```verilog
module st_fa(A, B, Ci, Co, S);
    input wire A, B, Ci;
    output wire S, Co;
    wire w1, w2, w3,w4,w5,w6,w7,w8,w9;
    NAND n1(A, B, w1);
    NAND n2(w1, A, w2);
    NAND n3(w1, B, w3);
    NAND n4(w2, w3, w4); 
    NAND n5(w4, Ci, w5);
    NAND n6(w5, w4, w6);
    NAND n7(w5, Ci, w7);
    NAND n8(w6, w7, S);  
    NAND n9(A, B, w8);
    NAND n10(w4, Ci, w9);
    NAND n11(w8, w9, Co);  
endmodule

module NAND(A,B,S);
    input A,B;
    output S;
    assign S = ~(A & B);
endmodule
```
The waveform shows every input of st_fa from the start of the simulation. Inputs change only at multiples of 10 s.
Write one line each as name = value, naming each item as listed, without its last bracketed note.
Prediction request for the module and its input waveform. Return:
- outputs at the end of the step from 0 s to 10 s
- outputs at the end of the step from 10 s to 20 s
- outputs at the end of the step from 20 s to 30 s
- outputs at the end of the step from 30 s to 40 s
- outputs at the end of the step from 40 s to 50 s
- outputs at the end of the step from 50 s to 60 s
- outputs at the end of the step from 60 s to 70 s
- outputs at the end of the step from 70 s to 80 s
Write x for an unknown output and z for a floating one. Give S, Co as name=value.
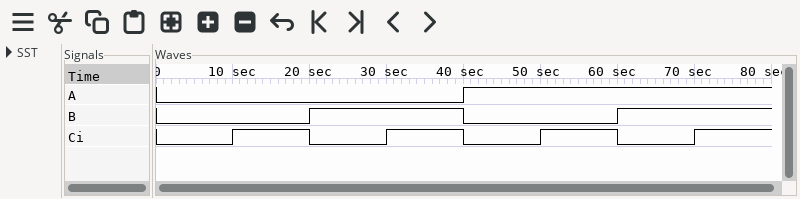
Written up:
outputs at the end of the step from 0 s to 10 s = S=0, Co=0
outputs at the end of the step from 10 s to 20 s = S=1, Co=0
outputs at the end of the step from 20 s to 30 s = S=1, Co=0
outputs at the end of the step from 30 s to 40 s = S=0, Co=1
outputs at the end of the step from 40 s to 50 s = S=1, Co=0
outputs at the end of the step from 50 s to 60 s = S=0, Co=1
outputs at the end of the step from 60 s to 70 s = S=0, Co=1
outputs at the end of the step from 70 s to 80 s = S=1, Co=1
